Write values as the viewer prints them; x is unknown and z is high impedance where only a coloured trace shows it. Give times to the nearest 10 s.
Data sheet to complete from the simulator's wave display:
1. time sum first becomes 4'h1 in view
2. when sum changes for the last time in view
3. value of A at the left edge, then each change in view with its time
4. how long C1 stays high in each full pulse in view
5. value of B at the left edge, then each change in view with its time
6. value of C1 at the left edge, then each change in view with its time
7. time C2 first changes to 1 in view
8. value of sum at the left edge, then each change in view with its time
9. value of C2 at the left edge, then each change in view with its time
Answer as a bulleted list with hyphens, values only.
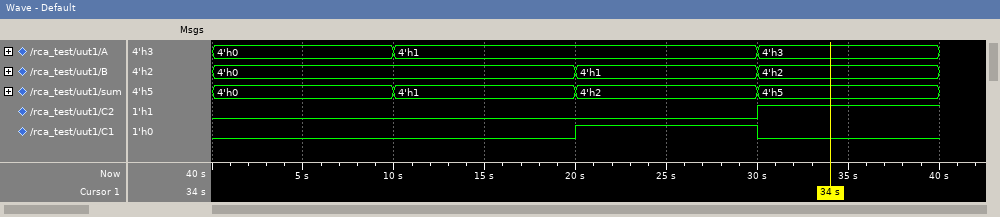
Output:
- 10 s
- 30 s
- 4'h0, 4'h1 at 10 s, 4'h3 at 30 s
- 10 s
- 4'h0, 4'h1 at 20 s, 4'h2 at 30 s
- 0, 1 at 20 s, 0 at 30 s
- 30 s
- 4'h0, 4'h1 at 10 s, 4'h2 at 20 s, 4'h5 at 30 s
- 0, 1 at 30 s
